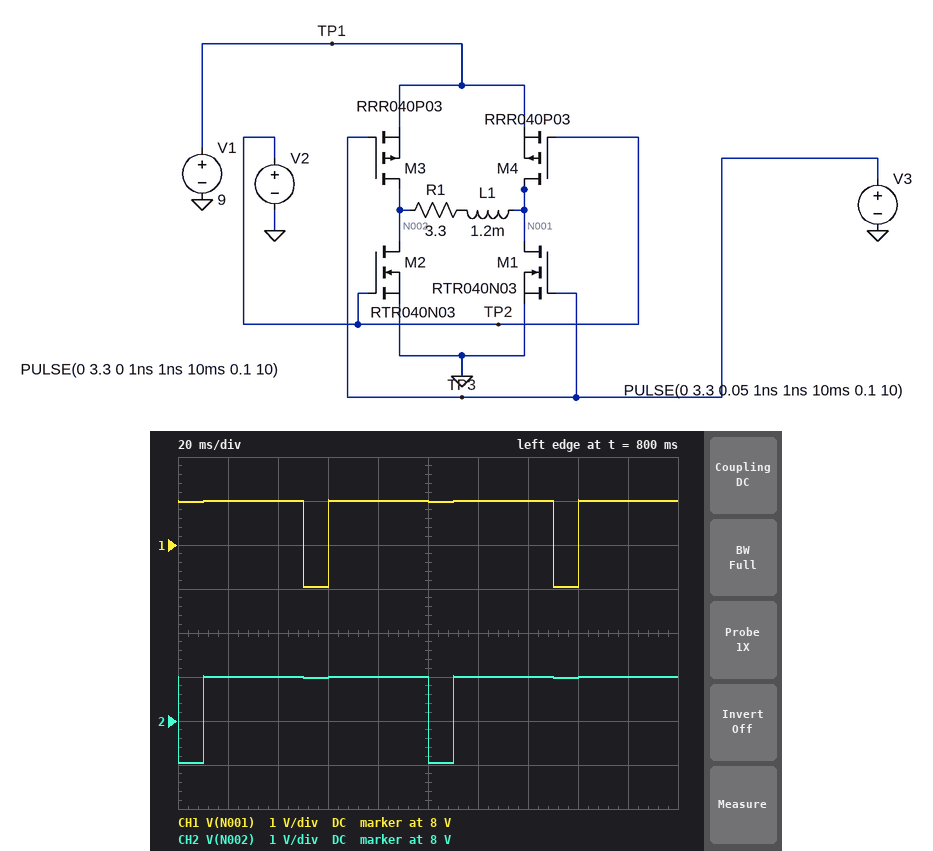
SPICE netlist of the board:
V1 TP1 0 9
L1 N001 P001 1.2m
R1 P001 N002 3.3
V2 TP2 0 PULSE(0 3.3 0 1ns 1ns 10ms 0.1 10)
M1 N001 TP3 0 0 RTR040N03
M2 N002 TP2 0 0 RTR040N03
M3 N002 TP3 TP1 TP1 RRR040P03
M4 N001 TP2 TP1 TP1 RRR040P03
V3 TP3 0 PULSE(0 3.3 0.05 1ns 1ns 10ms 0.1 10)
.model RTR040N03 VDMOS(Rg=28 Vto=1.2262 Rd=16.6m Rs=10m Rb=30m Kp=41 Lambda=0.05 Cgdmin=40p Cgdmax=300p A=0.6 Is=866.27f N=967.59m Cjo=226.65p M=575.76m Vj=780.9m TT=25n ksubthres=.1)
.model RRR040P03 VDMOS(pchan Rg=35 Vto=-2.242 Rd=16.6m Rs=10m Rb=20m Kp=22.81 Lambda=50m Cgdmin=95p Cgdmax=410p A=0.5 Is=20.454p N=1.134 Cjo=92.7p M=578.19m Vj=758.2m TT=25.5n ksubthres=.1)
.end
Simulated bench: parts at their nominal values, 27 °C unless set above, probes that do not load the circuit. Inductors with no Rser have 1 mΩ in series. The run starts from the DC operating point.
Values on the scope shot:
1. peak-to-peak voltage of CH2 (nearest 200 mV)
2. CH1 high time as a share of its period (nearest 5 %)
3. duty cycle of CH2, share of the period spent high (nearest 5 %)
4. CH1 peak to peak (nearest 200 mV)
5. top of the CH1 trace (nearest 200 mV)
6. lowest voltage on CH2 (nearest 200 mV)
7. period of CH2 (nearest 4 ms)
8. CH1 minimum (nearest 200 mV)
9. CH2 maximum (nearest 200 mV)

2.0 V
90 %
90 %
2.0 V
9.0 V
7.0 V
100 ms
7.0 V
9.0 V
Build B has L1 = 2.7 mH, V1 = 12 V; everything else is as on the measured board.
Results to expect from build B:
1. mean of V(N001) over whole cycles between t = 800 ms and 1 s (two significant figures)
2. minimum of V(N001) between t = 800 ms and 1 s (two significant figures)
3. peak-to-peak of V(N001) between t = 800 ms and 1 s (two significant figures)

12 V
10 V
2.0 V
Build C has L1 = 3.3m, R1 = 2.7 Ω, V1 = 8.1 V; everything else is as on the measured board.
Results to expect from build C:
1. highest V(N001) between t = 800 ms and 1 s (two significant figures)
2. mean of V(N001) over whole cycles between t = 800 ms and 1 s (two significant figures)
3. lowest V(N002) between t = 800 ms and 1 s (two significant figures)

8.1 V
7.9 V
6.1 V
